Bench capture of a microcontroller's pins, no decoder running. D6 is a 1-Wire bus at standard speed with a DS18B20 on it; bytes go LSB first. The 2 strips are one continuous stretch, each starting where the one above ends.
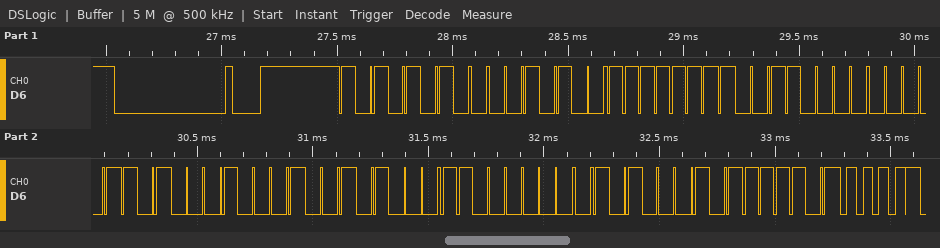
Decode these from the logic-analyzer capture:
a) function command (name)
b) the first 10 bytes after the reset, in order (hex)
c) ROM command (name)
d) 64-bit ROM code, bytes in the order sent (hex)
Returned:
Read Scratchpad
55 28 FF 0C B0 88 14 03 8A BE
Match ROM
28 FF 0C B0 88 14 03 8A
